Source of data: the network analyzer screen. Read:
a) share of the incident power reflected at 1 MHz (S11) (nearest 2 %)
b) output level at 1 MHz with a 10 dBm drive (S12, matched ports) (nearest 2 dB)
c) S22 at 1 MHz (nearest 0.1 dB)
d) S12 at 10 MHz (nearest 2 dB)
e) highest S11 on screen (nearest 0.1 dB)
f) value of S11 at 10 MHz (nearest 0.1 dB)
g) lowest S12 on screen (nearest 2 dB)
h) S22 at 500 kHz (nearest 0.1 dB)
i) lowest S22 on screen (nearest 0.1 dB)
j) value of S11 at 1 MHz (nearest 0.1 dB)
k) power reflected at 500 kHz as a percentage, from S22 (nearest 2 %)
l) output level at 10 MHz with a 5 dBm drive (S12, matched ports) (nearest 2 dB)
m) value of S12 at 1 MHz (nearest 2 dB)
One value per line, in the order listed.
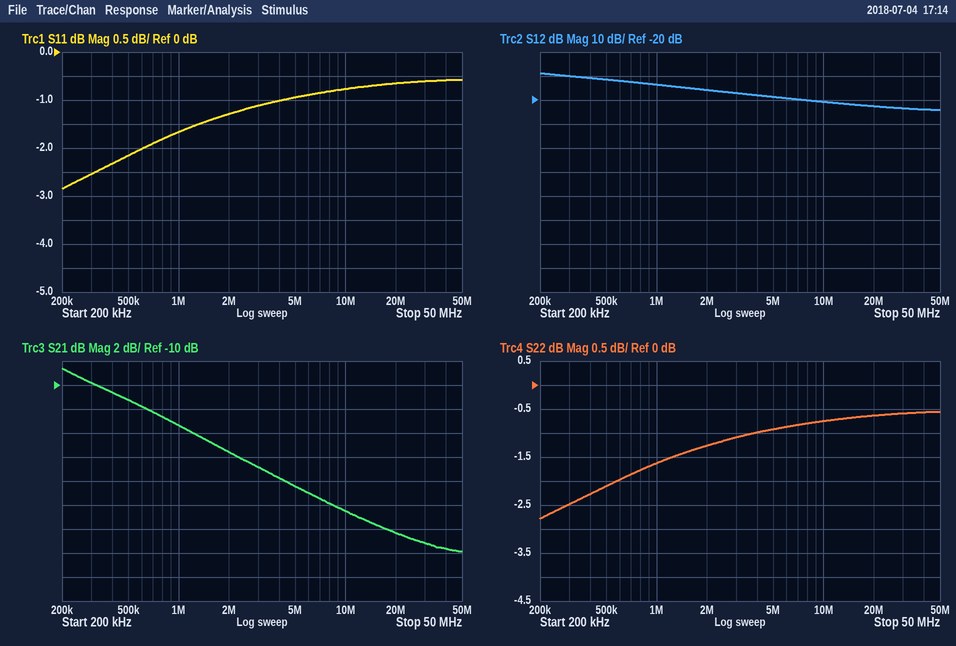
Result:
68 %
-4 dBm
-1.6 dB
-20 dB
-0.6 dB
-0.8 dB
-24 dB
-2.1 dB
-2.8 dB
-1.7 dB
62 %
-16 dBm
-14 dB
